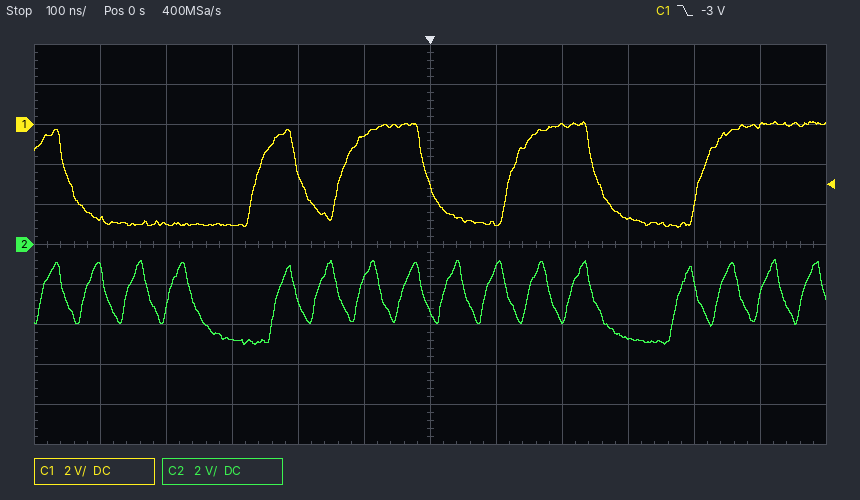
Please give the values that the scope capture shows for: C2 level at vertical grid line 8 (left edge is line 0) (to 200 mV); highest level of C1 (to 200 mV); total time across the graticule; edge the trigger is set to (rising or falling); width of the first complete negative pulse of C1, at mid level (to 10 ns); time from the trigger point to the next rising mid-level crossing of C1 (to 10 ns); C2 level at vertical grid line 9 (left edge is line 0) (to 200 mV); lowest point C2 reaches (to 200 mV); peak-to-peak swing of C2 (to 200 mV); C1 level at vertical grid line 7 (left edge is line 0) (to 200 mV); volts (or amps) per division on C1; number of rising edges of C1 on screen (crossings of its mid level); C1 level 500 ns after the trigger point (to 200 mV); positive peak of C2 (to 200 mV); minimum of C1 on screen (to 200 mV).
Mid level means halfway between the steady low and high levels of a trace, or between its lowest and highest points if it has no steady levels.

-3.8 V
200 mV
1.2 µs
falling
290 ns
120 ns
-4.6 V
-5.0 V
4.2 V
-5.0 V
2 V
4
0.0 V
-800 mV
-5.2 V
